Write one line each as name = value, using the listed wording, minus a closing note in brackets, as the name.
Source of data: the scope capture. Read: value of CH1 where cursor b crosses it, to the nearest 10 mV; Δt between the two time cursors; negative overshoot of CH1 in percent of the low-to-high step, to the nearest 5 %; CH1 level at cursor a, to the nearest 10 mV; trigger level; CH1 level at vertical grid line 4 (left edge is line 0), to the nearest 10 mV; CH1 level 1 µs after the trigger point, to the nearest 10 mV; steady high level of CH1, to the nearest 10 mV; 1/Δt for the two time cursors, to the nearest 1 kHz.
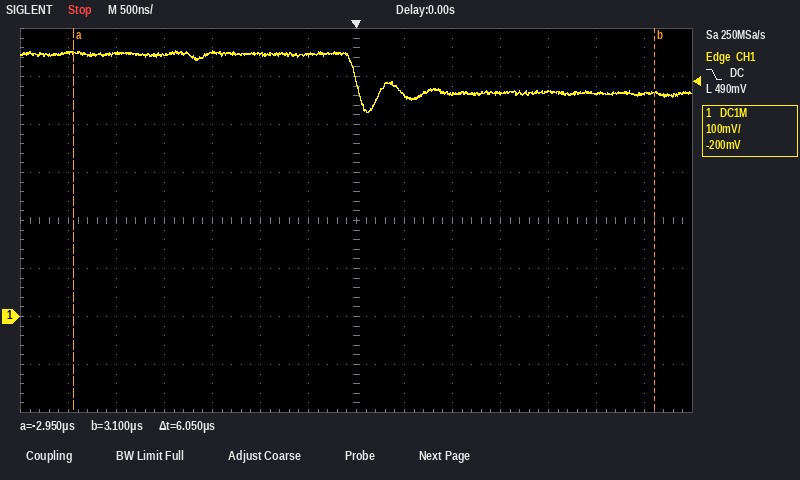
value of CH1 where cursor b crosses it, to the nearest 10 mV = 470 mV
Δt between the two time cursors = 6.05 µs
negative overshoot of CH1 in percent of the low-to-high step, to the nearest 5 % = 50 %
CH1 level at cursor a, to the nearest 10 mV = 550 mV
trigger level = 490 mV
CH1 level at vertical grid line 4 (left edge is line 0), to the nearest 10 mV = 550 mV
CH1 level 1 µs after the trigger point, to the nearest 10 mV = 460 mV
steady high level of CH1, to the nearest 10 mV = 550 mV
1/Δt for the two time cursors, to the nearest 1 kHz = 165 kHz
